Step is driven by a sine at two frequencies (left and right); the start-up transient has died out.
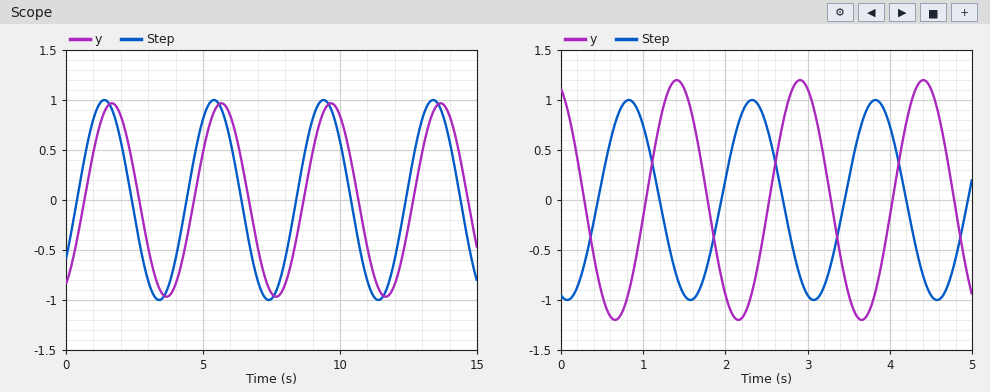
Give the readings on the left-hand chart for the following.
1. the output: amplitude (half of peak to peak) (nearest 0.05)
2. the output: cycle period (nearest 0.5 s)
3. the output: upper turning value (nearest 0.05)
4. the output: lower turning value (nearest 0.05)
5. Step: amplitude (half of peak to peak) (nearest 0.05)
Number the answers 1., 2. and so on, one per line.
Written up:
1. 0.95
2. 4.0 s
3. 0.95
4. -0.95
5. 1.00
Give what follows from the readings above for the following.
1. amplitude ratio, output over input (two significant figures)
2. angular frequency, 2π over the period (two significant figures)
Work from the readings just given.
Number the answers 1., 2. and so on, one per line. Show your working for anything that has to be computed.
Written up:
1. 0.95 / 1 = 0.95
2. 2π / 4 = 1.6 rad/s
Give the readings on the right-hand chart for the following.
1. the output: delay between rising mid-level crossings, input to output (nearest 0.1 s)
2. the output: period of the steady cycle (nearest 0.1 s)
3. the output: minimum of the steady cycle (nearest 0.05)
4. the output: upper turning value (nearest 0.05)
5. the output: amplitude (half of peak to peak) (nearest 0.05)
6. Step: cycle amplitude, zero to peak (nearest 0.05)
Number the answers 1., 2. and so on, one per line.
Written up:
1. 0.6 s
2. 1.5 s
3. -1.20
4. 1.20
5. 1.20
6. 1.00
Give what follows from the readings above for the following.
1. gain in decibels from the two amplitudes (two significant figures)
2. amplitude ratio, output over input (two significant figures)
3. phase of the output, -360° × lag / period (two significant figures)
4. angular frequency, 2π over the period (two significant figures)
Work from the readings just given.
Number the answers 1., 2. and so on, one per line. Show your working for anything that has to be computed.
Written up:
1. 20 log10(1.2 / 1) = 1.6 dB
2. 1.2 / 1 = 1.2
3. -360 × 0.6 / 1.5 = -140°
4. 2π / 1.5 = 4.2 rad/s
